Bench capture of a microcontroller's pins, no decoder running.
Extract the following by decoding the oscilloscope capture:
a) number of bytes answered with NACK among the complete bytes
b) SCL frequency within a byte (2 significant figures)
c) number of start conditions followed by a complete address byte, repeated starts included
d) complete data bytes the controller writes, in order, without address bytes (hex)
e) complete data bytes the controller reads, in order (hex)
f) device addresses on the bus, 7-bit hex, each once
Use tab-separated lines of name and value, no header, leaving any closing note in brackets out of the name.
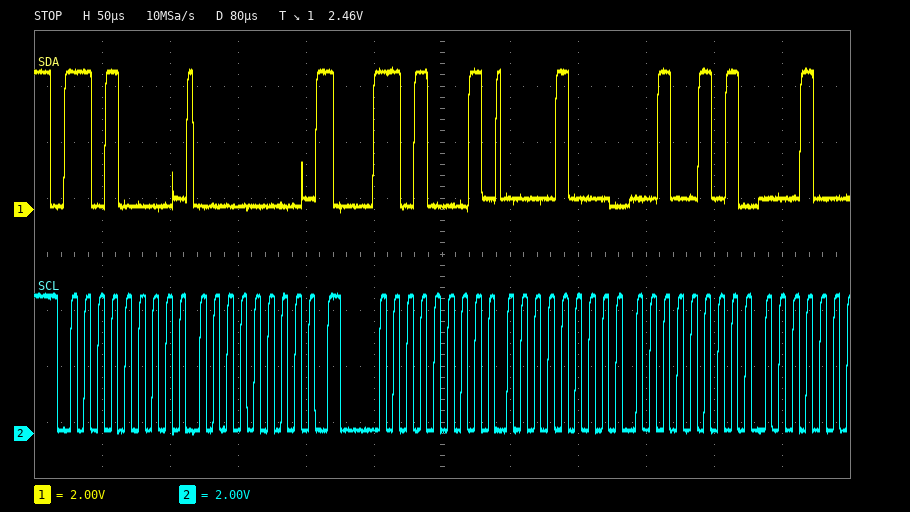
number of bytes answered with NACK among the complete bytes	0
SCL frequency within a byte	100 kHz
number of start conditions followed by a complete address byte, repeated starts included	2
complete data bytes the controller writes, in order, without address bytes	00
complete data bytes the controller reads, in order	08 25
device addresses on the bus, 7-bit hex, each once	0x68
